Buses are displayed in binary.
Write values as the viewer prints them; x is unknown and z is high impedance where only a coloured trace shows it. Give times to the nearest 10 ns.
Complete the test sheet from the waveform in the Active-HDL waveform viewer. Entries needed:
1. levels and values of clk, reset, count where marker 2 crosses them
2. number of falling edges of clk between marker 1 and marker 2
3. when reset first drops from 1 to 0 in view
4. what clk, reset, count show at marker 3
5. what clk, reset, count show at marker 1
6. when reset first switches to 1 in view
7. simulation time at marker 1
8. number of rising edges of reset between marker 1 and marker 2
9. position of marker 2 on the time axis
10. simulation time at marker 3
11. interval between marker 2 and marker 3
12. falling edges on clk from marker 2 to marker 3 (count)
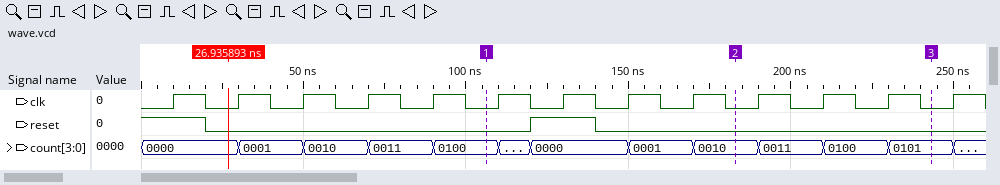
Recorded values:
clk=0, reset=0, count=0010
4
20 ns
clk=0, reset=0, count=0101
clk=0, reset=0, count=0100
120 ns
110 ns
1
180 ns
240 ns
60 ns
3
